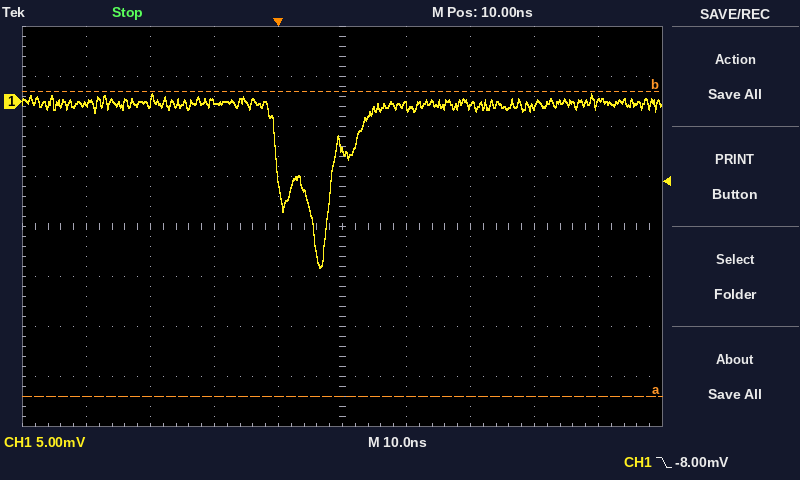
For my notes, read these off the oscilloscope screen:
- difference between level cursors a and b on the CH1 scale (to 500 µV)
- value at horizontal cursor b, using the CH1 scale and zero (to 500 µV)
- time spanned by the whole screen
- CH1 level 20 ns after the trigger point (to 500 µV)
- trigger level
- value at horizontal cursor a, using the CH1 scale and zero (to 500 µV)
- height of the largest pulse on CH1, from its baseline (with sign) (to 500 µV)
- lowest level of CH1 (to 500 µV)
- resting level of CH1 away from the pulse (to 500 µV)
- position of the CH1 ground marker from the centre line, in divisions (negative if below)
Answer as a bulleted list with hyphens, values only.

- 30.5 mV
- 1.0 mV
- 100 ns
- -500 µV
- -8.00 mV
- -29.5 mV
- -16.5 mV
- -16.5 mV
- 0.0 mV
- +2.5 div
